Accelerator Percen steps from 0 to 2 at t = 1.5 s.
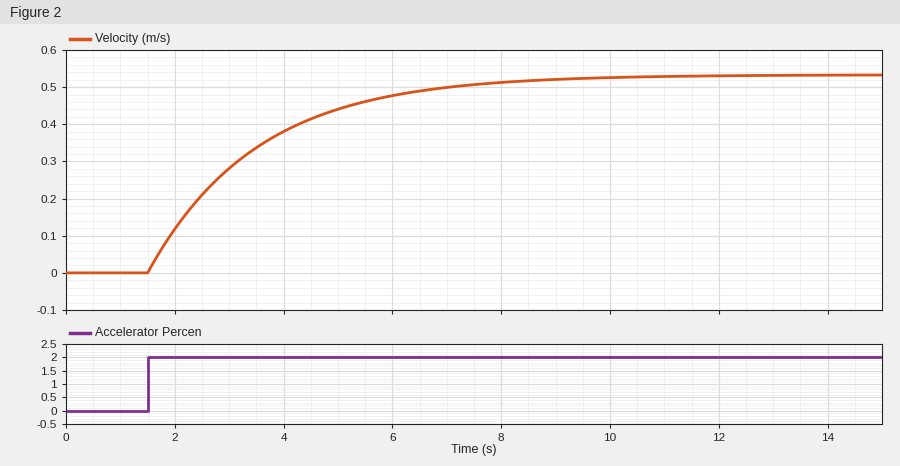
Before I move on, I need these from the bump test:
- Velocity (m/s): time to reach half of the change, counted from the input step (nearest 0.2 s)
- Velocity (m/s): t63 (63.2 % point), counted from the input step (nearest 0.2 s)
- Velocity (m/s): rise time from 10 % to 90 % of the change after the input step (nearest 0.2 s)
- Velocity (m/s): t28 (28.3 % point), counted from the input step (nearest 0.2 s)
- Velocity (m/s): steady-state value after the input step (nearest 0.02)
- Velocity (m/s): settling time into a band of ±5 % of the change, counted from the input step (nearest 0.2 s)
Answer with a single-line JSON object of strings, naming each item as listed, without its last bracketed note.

{"Velocity (m/s): time to reach half of the change, counted from the input step": "1.4 s", "Velocity (m/s): t63 (63.2 % point), counted from the input step": "2.0 s", "Velocity (m/s): rise time from 10 % to 90 % of the change after the input step": "4.4 s", "Velocity (m/s): t28 (28.3 % point), counted from the input step": "0.6 s", "Velocity (m/s): steady-state value after the input step": "0.54", "Velocity (m/s): settling time into a band of ±5 % of the change, counted from the input step": "6.0 s"}
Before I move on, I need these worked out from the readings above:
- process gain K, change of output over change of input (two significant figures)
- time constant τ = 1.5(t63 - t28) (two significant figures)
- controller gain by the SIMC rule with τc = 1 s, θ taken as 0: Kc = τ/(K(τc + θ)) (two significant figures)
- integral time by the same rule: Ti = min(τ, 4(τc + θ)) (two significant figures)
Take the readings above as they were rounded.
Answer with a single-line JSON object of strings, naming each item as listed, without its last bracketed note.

{"process gain K, change of output over change of input": "0.27", "time constant τ = 1.5(t63 - t28)": "2.1 s", "controller gain by the SIMC rule with τc = 1 s, θ taken as 0: Kc = τ/(K(τc + θ))": "7.8", "integral time by the same rule: Ti = min(τ, 4(τc + θ))": "2.1 s"}
